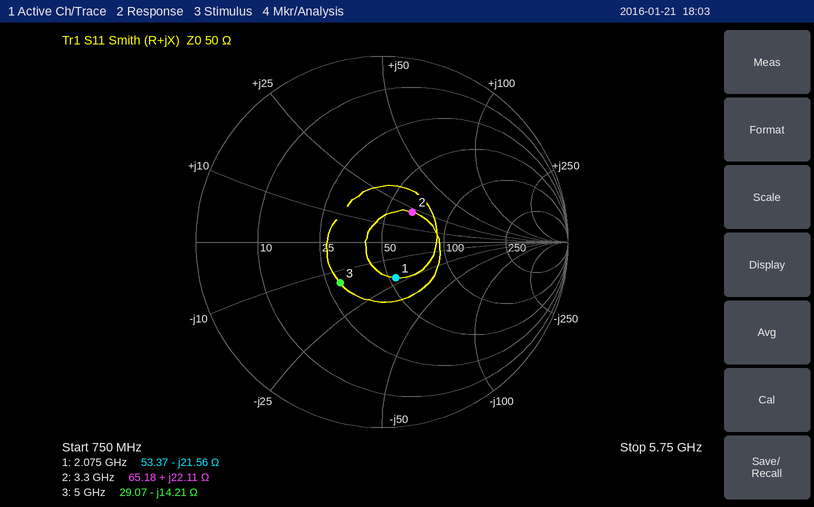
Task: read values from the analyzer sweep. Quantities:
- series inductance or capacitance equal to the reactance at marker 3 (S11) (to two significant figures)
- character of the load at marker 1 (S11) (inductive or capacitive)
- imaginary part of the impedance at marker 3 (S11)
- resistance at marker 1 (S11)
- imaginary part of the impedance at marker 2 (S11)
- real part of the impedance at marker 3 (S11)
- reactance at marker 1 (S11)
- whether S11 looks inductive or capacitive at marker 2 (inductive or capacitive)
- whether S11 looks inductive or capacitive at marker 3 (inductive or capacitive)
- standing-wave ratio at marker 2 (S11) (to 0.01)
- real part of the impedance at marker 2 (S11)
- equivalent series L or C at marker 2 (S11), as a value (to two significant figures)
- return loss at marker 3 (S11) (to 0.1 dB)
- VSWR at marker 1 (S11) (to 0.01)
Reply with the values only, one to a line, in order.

2.2 pF
capacitive
-14.21 Ω
53.37 Ω
+22.11 Ω
29.07 Ω
-21.56 Ω
inductive
capacitive
1.59
65.18 Ω
1.1 nH
10.0 dB
1.52
